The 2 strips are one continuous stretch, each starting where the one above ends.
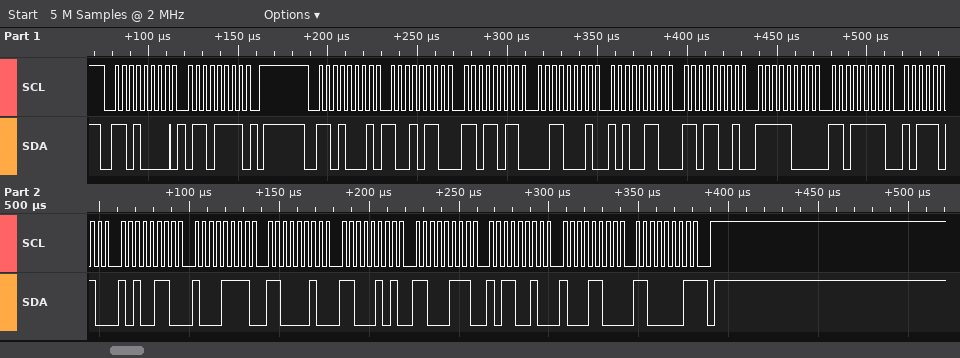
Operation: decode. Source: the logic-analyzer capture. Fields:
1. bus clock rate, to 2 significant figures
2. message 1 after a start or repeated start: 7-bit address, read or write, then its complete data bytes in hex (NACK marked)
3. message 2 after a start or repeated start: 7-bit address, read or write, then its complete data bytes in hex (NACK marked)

250 kHz
0x68 write: 6F
0x68 read: 96 DB 31 A6 D9 F8 DF BA A6 8F C2 C5 C7 B2 8C C1 NACK
